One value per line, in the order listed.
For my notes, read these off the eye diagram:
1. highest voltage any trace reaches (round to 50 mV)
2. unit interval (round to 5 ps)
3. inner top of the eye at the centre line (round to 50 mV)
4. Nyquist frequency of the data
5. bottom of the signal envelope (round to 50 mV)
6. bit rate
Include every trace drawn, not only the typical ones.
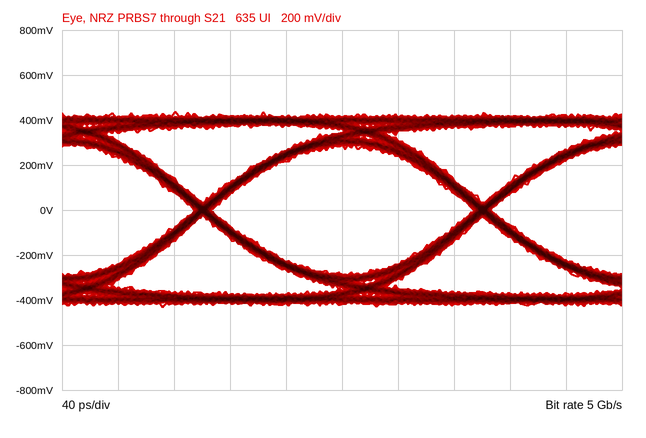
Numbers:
450 mV
200 ps
300 mV
2.5 GHz
-450 mV
5 Gb/s
